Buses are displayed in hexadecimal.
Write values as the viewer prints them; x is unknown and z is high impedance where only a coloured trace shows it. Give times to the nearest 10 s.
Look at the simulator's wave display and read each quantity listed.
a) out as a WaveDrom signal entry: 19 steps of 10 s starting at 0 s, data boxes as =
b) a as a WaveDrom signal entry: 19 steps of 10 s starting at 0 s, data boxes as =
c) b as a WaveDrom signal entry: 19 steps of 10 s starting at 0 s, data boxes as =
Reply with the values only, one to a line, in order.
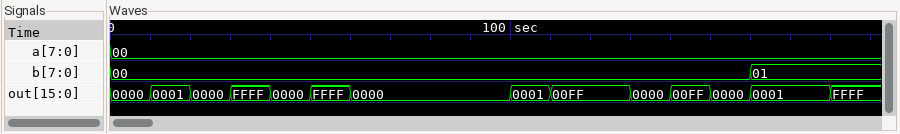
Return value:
{name: 'out', wave: '=======...==.====.=', data: '0000 0001 0000 FFFF 0000 FFFF 0000 0001 00FF 0000 00FF 0000 0001 FFFF'}
{name: 'a', wave: '=..................', data: '00'}
{name: 'b', wave: '=...............=..', data: '00 01'}
